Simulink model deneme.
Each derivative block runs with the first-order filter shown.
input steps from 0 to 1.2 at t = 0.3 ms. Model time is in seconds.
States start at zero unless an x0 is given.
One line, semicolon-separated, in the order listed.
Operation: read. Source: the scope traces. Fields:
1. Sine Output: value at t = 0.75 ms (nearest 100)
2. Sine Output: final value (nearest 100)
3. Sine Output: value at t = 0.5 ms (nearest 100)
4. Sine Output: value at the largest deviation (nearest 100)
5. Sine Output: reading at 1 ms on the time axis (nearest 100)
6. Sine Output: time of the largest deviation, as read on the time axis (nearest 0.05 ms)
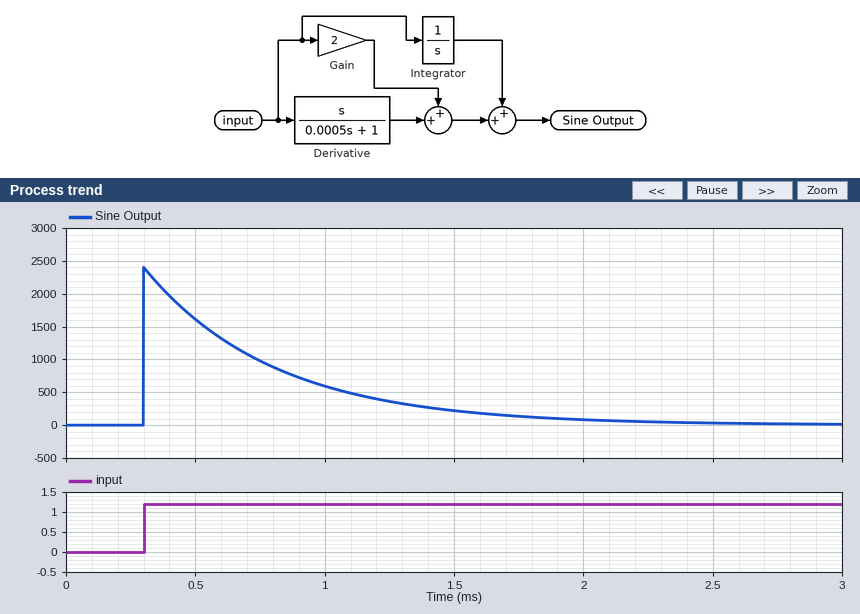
1000; 0; 1600; 2400; 600; 0.30 ms
